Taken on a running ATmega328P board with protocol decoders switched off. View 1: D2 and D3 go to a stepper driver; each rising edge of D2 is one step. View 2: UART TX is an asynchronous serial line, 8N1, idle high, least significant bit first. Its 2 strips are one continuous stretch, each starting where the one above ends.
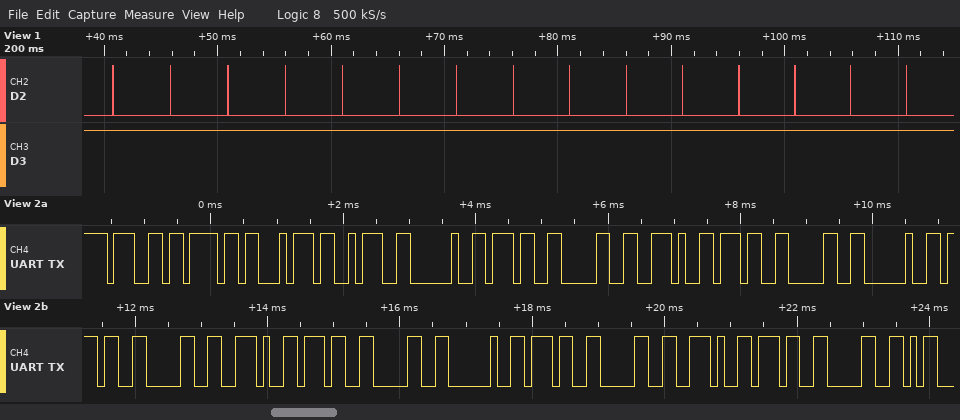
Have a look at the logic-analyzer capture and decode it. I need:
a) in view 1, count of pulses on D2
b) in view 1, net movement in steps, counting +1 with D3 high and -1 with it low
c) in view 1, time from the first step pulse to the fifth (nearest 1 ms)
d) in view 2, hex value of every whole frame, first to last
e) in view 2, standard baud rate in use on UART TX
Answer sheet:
15
+15
20 ms
0x67 0x6F 0x74 0x3A 0x20 0x37 0x30 0x2E 0x37 0x30 0x20 0x37 0x30 0x2E 0x37 0x30 0x20 0x37 0x30 0x2E 0x37 0x30
9600 baud
